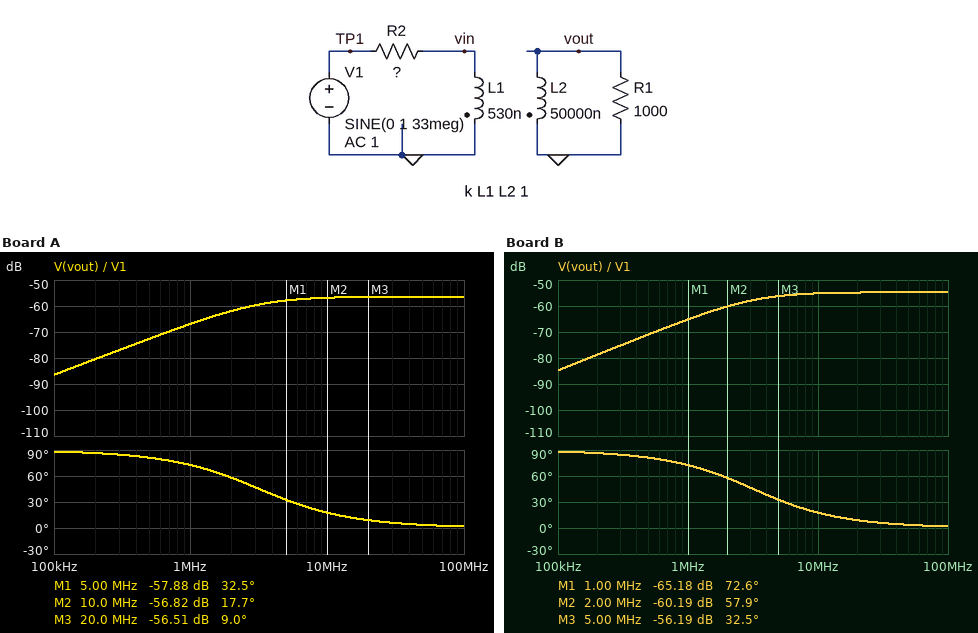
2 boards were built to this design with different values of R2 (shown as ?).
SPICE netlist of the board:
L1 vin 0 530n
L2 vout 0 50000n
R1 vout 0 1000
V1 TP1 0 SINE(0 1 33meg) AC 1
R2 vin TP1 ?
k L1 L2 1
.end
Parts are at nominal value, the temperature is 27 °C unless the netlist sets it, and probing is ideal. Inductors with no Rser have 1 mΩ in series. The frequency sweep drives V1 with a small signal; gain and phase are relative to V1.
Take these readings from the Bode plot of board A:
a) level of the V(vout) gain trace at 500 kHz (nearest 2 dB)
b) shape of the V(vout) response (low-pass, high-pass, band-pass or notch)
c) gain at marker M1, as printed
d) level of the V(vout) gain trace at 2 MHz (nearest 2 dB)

-72 dB
high-pass
-57.88 dB
-62 dB
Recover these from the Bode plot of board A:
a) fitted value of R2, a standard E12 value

68 kΩ
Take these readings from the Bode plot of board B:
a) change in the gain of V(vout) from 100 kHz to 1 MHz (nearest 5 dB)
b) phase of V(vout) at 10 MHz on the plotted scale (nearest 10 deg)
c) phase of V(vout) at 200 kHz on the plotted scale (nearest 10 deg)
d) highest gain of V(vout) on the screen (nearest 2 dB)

20 dB
20 deg
90 deg
-54 dB
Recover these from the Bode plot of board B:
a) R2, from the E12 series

56 kΩ
